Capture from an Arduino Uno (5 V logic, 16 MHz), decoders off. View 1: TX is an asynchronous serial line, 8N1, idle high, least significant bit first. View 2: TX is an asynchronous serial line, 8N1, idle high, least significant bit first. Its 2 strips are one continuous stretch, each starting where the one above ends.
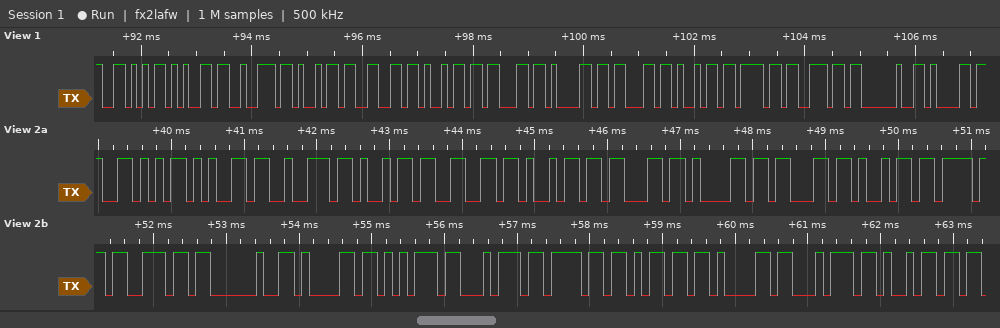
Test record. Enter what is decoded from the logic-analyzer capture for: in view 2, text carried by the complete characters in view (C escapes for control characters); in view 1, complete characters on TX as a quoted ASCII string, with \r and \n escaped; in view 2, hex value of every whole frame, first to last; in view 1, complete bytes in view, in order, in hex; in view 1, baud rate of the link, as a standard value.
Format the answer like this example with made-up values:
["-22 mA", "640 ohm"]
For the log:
["\"Verificacion automati\"", "\"Verificacion a\"", "0x56 0x65 0x72 0x69 0x66 0x69 0x63 0x61 0x63 0x69 0x6F 0x6E 0x20 0x61 0x75 0x74 0x6F 0x6D 0x61 0x74 0x69", "56 65 72 69 66 69 63 61 63 69 6F 6E 20 61", "9600 baud"]
